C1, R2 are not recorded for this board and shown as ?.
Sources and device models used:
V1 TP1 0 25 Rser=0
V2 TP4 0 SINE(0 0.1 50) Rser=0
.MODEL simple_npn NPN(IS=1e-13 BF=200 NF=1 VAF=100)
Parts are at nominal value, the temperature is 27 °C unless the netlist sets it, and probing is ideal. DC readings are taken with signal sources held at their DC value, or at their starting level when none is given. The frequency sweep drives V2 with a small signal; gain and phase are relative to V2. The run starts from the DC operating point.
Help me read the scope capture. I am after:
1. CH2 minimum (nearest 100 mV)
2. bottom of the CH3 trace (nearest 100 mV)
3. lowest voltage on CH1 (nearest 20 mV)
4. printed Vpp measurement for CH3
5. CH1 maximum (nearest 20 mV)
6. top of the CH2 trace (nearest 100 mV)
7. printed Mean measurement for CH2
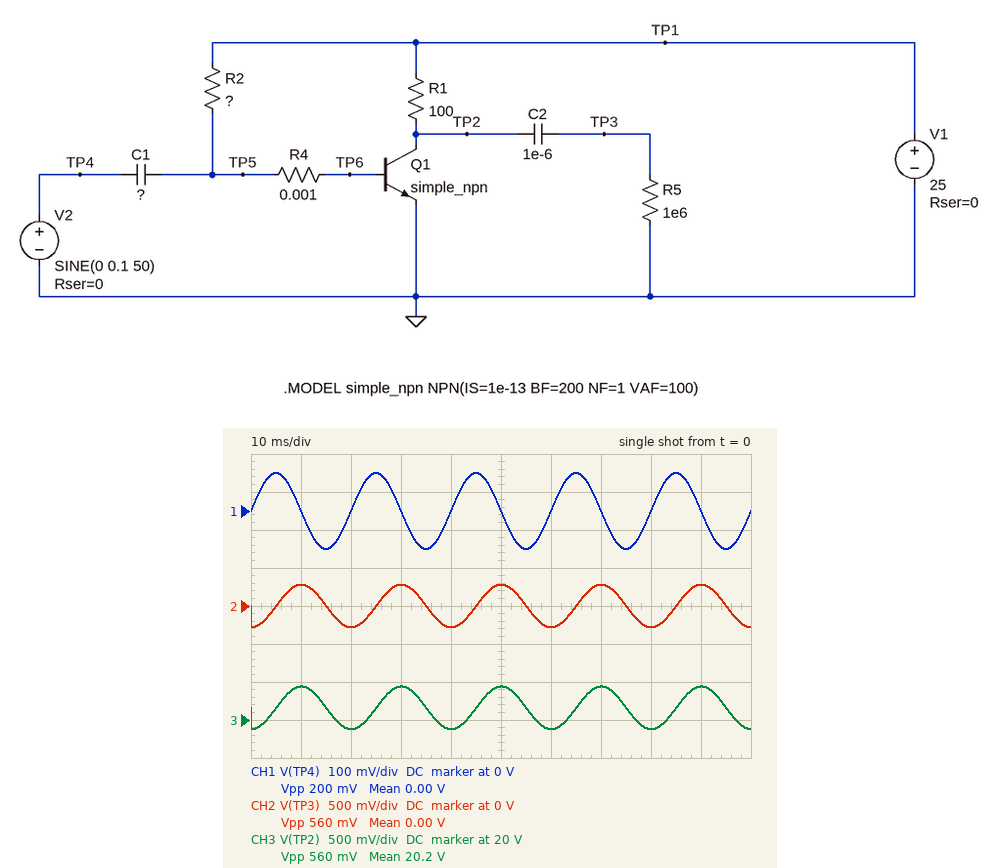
-300 mV
19.9 V
-100 mV
560 mV
100 mV
300 mV
0.00 V
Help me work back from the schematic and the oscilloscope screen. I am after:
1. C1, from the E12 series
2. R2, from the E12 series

390 nF
120 kΩ
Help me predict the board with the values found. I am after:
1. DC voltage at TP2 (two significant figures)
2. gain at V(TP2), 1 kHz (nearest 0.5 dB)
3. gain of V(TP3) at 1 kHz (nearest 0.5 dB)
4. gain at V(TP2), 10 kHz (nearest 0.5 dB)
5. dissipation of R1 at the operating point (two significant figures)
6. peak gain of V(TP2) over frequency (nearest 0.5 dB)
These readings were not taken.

20 V
34.5 dB
34.5 dB
44.5 dB
230 mW
45.0 dB
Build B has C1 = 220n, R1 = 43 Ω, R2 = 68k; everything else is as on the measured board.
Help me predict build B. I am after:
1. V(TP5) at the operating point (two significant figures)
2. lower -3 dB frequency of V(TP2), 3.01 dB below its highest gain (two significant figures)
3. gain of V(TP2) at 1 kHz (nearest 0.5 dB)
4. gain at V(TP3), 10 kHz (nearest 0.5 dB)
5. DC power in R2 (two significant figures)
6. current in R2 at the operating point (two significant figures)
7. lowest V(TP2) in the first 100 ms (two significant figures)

710 mV
10 kHz
23.0 dB
40.0 dB
8.7 mW
360 µA
21 V
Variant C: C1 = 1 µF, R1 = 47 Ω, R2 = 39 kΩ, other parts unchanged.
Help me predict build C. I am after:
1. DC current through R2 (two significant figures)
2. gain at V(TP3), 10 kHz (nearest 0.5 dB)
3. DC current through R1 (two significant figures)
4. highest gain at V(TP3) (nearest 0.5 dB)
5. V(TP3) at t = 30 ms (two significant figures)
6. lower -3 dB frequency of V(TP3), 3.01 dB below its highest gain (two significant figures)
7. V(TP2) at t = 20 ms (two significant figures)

620 µA
47.5 dB
150 mA
48.0 dB
330 mV
3.8 kHz
18 V
